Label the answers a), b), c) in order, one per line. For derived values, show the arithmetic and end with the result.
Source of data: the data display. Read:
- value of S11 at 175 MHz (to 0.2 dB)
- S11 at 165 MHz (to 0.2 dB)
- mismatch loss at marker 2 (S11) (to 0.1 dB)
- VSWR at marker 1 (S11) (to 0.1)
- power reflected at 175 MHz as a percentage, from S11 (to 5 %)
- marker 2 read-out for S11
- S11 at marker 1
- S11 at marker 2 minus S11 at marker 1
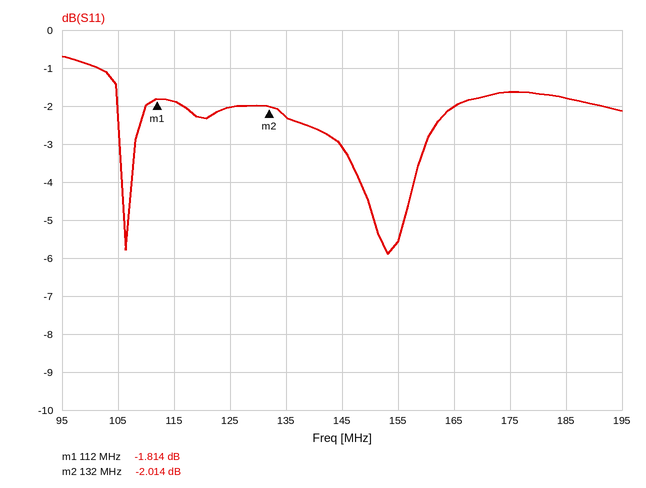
a) -1.6 dB
b) -2.0 dB
c) −10 log10(1 − 10^(-2.014/10)) ≈ 4.3 dB
d) (1 + 0.8115)/(1 − 0.8115) ≈ 9.6
e) 10^(-1.6/10) ≈ 69.2 %, so 70 % to the nearest 5 %
f) -2.014 dB
g) -1.814 dB
h) -2.014 − (-1.814) = -0.200 dB
